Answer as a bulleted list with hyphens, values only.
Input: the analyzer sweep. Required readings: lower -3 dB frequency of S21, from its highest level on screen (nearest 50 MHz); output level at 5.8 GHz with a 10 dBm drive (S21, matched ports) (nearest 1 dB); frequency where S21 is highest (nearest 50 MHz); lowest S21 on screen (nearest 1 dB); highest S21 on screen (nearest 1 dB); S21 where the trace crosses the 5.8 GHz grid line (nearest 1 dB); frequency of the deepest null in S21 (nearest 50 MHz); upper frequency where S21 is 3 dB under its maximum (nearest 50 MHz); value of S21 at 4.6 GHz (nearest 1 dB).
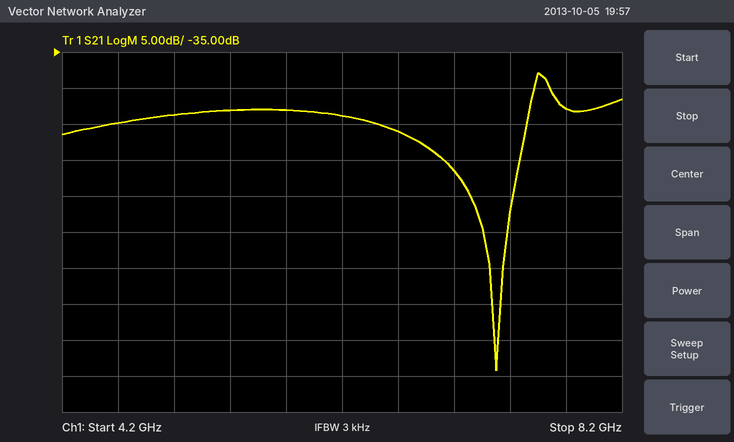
- 7.55 GHz
- -33 dBm
- 7.60 GHz
- -79 dB
- -38 dB
- -43 dB
- 7.30 GHz
- 7.70 GHz
- -45 dB
